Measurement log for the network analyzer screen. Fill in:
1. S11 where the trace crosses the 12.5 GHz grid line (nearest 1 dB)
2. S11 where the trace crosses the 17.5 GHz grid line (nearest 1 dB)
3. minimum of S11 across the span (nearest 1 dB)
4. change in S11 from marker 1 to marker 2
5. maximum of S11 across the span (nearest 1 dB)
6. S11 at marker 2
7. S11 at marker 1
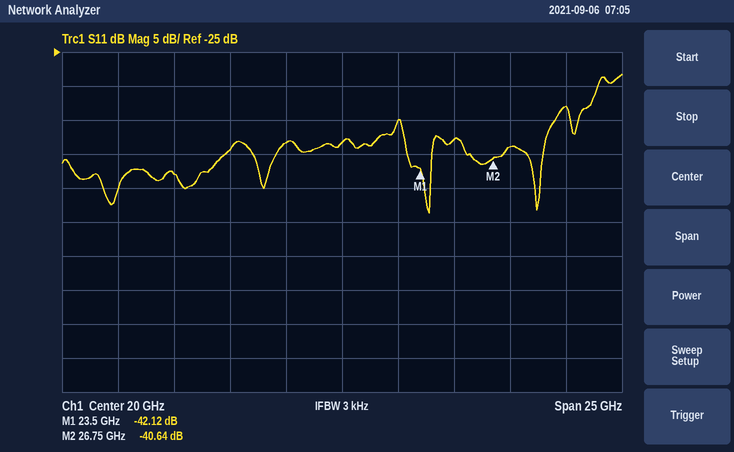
-43 dB
-38 dB
-49 dB
1.48 dB
-28 dB
-40.64 dB
-42.12 dB
